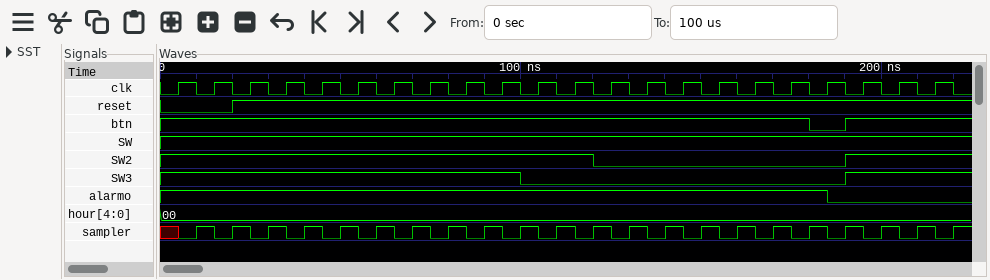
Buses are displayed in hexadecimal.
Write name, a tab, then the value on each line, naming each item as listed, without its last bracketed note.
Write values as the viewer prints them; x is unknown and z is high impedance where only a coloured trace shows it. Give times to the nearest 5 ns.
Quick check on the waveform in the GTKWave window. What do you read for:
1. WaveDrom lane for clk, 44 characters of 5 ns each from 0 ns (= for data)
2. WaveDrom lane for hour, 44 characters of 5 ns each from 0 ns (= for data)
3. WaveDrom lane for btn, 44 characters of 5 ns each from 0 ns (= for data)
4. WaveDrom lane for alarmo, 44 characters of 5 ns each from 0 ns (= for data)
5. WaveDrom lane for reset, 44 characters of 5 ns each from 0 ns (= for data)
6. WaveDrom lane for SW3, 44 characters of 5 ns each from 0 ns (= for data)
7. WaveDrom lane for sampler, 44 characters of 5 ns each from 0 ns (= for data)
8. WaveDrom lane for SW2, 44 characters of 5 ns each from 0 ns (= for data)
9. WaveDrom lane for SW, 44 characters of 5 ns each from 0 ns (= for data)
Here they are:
WaveDrom lane for clk, 44 characters of 5 ns each from 0 ns	{name: 'clk', wave: '01010101010101010101010101010101010101010101'}
WaveDrom lane for hour, 44 characters of 5 ns each from 0 ns	{name: 'hour', wave: '=...........................................', data: '00'}
WaveDrom lane for btn, 44 characters of 5 ns each from 0 ns	{name: 'btn', wave: '1...................................0.1.....'}
WaveDrom lane for alarmo, 44 characters of 5 ns each from 0 ns	{name: 'alarmo', wave: '1....................................0......'}
WaveDrom lane for reset, 44 characters of 5 ns each from 0 ns	{name: 'reset', wave: '0...1.......................................'}
WaveDrom lane for SW3, 44 characters of 5 ns each from 0 ns	{name: 'SW3', wave: '1...................0.................1.....'}
WaveDrom lane for sampler, 44 characters of 5 ns each from 0 ns	{name: 'sampler', wave: 'x0101010101010101010101010101010101010101010'}
WaveDrom lane for SW2, 44 characters of 5 ns each from 0 ns	{name: 'SW2', wave: '1.......................0.............1.....'}
WaveDrom lane for SW, 44 characters of 5 ns each from 0 ns	{name: 'SW', wave: '1...........................................'}
